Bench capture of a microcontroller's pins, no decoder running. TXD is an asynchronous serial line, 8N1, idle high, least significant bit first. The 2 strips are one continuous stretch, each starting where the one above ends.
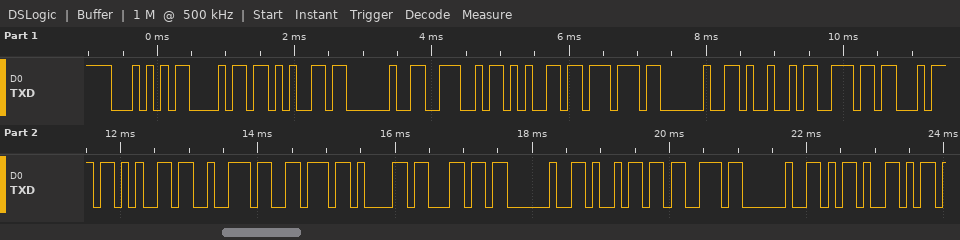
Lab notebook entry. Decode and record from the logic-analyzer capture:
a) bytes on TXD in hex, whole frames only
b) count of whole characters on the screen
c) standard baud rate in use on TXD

54 68 65 20 4E 65 77 20 49 6E 74 65 72 76 61 6C 20 69 73 20 2D
21
9600 baud
